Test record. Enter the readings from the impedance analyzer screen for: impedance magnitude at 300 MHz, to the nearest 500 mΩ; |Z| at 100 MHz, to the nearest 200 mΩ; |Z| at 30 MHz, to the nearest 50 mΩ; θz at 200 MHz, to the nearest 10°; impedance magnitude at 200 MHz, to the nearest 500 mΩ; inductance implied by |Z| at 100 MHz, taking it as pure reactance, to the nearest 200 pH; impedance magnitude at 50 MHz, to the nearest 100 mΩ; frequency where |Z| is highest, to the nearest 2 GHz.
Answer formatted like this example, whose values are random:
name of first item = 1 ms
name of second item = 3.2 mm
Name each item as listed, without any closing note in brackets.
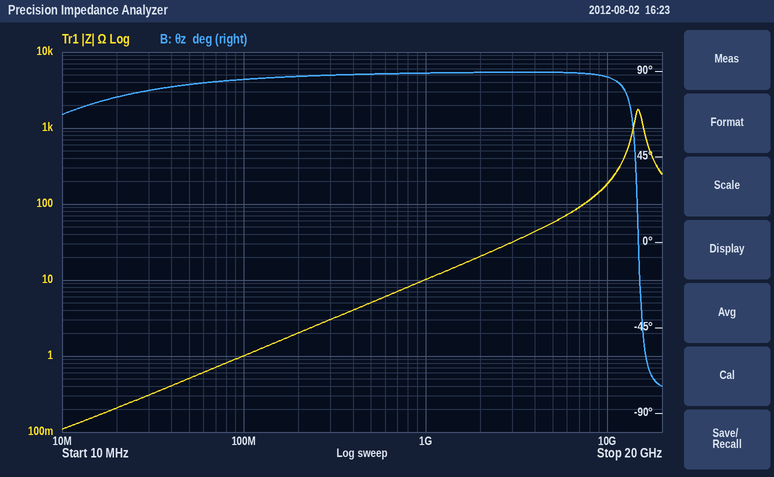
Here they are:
impedance magnitude at 300 MHz, to the nearest 500 mΩ = 3.0 Ω
|Z| at 100 MHz, to the nearest 200 mΩ = 1.0 Ω
|Z| at 30 MHz, to the nearest 50 mΩ = 300 mΩ
θz at 200 MHz, to the nearest 10° = 90°
impedance magnitude at 200 MHz, to the nearest 500 mΩ = 2.0 Ω
inductance implied by |Z| at 100 MHz, taking it as pure reactance, to the nearest 200 pH = 1.6 nH
impedance magnitude at 50 MHz, to the nearest 100 mΩ = 500 mΩ
frequency where |Z| is highest, to the nearest 2 GHz = 14 GHz
